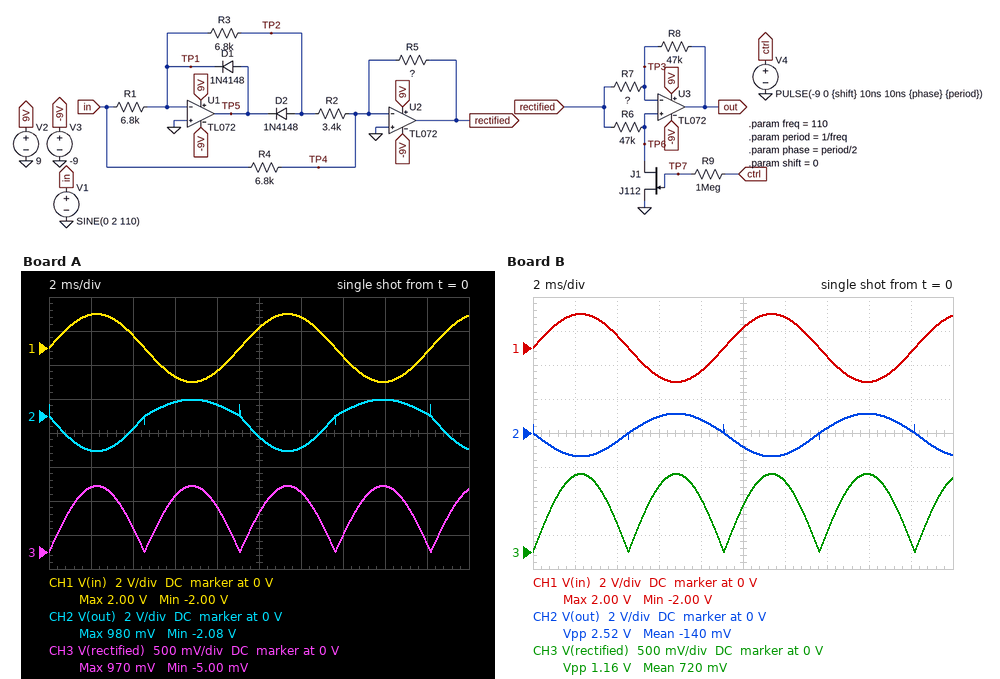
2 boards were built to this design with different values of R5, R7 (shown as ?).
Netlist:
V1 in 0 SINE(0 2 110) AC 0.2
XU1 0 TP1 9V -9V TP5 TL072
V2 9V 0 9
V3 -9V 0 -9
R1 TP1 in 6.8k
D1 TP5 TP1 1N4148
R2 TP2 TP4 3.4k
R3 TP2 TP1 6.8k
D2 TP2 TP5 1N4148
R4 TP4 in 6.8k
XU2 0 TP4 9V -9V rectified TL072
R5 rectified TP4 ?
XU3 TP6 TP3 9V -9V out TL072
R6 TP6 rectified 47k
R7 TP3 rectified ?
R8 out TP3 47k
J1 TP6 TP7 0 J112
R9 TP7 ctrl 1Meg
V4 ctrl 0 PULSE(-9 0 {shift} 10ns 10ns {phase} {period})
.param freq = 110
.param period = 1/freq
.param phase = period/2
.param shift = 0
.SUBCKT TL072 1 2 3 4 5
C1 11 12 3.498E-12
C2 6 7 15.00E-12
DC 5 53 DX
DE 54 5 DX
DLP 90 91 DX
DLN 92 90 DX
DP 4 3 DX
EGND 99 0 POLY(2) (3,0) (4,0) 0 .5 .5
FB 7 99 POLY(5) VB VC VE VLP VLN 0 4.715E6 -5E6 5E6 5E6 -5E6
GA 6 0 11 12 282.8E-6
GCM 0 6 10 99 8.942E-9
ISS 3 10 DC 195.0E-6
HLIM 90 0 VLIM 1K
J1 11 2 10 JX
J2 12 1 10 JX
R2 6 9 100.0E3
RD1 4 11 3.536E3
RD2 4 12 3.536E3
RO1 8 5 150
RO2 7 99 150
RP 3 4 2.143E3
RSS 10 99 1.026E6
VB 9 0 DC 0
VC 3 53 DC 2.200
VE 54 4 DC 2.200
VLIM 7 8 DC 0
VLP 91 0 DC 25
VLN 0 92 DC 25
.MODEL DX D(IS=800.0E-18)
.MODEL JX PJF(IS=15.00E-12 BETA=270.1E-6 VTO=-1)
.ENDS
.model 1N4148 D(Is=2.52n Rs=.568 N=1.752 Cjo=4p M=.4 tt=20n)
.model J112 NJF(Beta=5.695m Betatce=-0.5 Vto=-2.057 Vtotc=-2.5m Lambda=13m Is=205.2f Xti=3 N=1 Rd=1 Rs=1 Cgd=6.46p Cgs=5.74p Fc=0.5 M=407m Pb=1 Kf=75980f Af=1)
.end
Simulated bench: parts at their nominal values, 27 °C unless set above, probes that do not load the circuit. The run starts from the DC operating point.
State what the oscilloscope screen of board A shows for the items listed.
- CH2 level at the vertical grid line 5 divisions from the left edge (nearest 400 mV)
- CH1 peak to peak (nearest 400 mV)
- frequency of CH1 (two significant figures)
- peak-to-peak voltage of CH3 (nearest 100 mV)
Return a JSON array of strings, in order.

["-1.2 V", "4.0 V", "110 Hz", "1.0 V"]
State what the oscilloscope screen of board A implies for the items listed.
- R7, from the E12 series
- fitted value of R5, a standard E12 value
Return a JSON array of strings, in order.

["22 kΩ", "3.3 kΩ"]
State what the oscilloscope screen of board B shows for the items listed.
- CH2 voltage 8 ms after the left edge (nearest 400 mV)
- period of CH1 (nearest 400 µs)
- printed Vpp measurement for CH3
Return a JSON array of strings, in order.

["800 mV", "9.2 ms", "1.16 V"]
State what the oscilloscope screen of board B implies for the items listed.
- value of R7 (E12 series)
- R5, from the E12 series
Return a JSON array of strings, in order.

["39 kΩ", "3.9 kΩ"]
